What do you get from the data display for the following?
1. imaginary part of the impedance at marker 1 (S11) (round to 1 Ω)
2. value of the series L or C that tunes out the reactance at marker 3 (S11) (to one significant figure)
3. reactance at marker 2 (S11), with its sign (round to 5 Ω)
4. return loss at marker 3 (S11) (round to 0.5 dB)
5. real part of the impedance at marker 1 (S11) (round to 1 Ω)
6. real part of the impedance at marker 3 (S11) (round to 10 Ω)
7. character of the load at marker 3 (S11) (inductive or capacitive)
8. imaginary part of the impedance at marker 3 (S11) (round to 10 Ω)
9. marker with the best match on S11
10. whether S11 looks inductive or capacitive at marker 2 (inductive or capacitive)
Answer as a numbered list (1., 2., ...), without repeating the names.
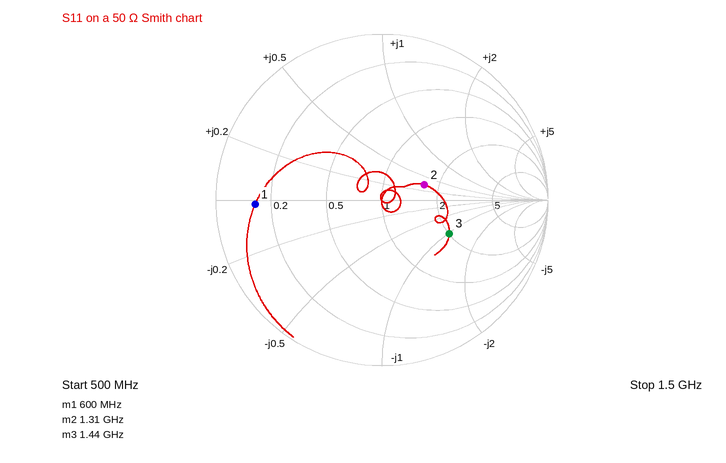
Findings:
1. -1 Ω
2. 6 nH
3. +15 Ω
4. 7.0 dB
5. 7 Ω
6. 100 Ω
7. capacitive
8. -50 Ω
9. marker 2
10. inductive
